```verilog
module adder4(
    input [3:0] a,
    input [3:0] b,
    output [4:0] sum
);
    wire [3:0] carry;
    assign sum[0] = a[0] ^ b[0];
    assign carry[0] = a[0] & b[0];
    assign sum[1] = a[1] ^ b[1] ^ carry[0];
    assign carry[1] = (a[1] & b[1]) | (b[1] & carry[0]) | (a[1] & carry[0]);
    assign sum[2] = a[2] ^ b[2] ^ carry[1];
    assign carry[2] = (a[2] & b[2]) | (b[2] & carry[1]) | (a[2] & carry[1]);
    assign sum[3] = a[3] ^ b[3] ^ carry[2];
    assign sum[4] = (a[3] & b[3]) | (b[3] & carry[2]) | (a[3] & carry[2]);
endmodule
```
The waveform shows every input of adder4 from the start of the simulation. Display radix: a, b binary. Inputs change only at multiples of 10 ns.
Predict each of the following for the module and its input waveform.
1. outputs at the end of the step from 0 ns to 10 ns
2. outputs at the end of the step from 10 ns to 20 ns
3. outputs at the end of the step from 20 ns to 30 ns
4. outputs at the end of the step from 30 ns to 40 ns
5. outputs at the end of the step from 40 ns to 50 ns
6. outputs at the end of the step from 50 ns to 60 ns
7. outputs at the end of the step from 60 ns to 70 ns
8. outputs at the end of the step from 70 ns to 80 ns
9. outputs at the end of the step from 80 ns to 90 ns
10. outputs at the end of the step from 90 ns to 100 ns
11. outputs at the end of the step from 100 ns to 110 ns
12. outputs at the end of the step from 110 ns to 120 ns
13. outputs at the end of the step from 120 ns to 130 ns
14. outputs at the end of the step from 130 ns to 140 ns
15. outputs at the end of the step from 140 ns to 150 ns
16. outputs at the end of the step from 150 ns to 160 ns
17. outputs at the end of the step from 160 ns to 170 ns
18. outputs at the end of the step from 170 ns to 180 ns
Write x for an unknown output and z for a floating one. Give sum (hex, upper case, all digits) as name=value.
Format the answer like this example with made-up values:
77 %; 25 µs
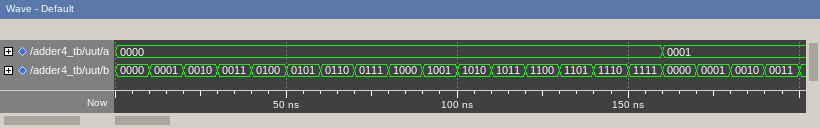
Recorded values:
sum=00; sum=01; sum=02; sum=03; sum=04; sum=05; sum=06; sum=07; sum=08; sum=09; sum=0A; sum=0B; sum=0C; sum=0D; sum=0E; sum=0F; sum=01; sum=02
